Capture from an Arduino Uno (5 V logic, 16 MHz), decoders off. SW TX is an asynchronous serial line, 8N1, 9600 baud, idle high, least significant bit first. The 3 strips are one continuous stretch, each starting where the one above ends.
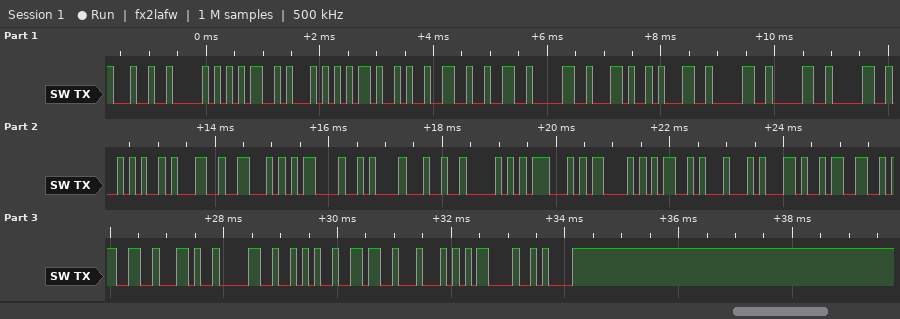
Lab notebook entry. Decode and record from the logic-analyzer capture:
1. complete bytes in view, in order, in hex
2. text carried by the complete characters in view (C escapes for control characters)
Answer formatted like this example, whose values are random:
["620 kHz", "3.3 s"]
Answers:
["24 50 4D 54 4B 32 32 30 2C 31 30 30 30 2A 31 46 0D 0A 24 50 47 43 4D 44 2C 33 33 2C 30 2A 36 44 0D 0A", "\"$PMTK220,1000*1F\\r\\n$PGCMD,33,0*6D\\r\\n\""]
